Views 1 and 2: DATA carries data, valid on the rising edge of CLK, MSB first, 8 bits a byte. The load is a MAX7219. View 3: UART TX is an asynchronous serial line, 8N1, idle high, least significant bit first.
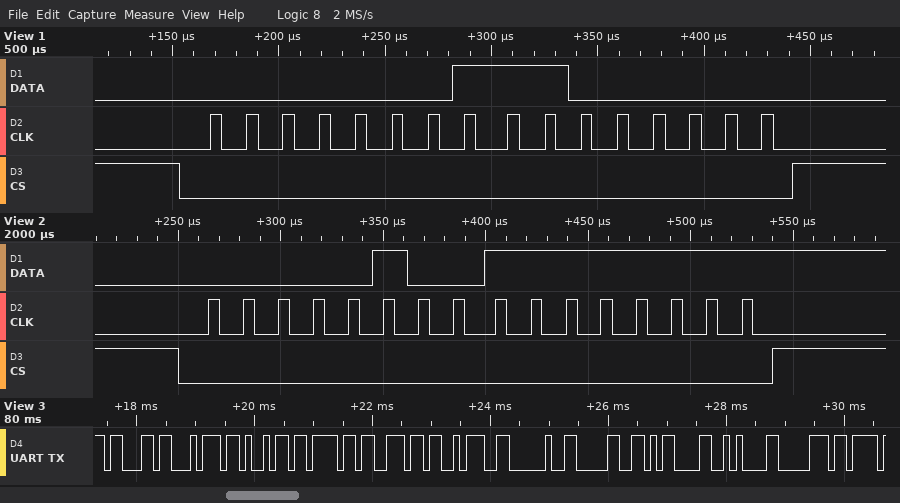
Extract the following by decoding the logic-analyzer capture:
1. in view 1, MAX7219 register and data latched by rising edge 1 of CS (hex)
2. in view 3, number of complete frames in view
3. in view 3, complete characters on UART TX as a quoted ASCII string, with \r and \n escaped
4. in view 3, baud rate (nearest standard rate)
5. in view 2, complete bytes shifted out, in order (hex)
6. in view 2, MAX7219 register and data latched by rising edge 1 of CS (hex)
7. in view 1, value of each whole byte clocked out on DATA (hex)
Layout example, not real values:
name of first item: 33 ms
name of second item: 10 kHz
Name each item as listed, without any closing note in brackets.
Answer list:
in view 1, MAX7219 register and data latched by rising edge 1 of CS: register 0x1, data 0xC0
in view 3, number of complete frames in view: 11
in view 3, complete characters on UART TX as a quoted ASCII string, with \r and \n escaped: "ction: 0\r\np"
in view 3, baud rate: 9600 baud
in view 2, complete bytes shifted out, in order: 04 FF
in view 2, MAX7219 register and data latched by rising edge 1 of CS: register 0x4, data 0xFF
in view 1, value of each whole byte clocked out on DATA: 01 C0
